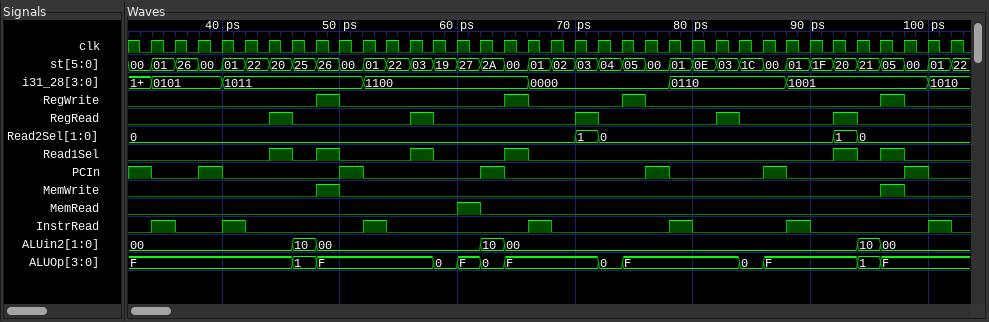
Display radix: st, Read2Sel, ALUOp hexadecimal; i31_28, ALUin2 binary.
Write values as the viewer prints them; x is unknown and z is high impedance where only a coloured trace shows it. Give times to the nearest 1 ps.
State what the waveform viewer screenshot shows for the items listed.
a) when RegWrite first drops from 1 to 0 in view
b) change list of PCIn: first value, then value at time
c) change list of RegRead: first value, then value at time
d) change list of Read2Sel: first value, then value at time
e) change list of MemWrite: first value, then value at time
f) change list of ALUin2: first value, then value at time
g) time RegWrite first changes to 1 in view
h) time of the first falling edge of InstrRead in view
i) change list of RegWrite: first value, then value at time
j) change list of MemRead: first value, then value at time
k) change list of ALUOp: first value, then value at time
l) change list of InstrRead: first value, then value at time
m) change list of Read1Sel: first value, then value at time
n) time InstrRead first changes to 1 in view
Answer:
50 ps
1, 0 at 34 ps, 1 at 38 ps, 0 at 40 ps, 1 at 50 ps, 0 at 52 ps, 1 at 62 ps, 0 at 64 ps, 1 at 76 ps, 0 at 78 ps, 1 at 86 ps, 0 at 88 ps, 1 at 98 ps, 0 at 100 ps
0, 1 at 44 ps, 0 at 46 ps, 1 at 56 ps, 0 at 58 ps, 1 at 70 ps, 0 at 72 ps, 1 at 82 ps, 0 at 84 ps, 1 at 92 ps, 0 at 94 ps
0, 1 at 70 ps, 0 at 72 ps, 1 at 92 ps, 0 at 94 ps
0, 1 at 48 ps, 0 at 50 ps, 1 at 96 ps, 0 at 98 ps
00, 10 at 46 ps, 00 at 48 ps, 10 at 62 ps, 00 at 64 ps, 10 at 94 ps, 00 at 96 ps
48 ps
36 ps
0, 1 at 48 ps, 0 at 50 ps, 1 at 64 ps, 0 at 66 ps, 1 at 74 ps, 0 at 76 ps, 1 at 96 ps, 0 at 98 ps
0, 1 at 60 ps, 0 at 62 ps
F, 1 at 46 ps, F at 48 ps, 0 at 58 ps, F at 60 ps, 0 at 62 ps, F at 64 ps, 0 at 72 ps, F at 74 ps, 0 at 84 ps, F at 86 ps, 1 at 94 ps, F at 96 ps
0, 1 at 34 ps, 0 at 36 ps, 1 at 40 ps, 0 at 42 ps, 1 at 52 ps, 0 at 54 ps, 1 at 66 ps, 0 at 68 ps, 1 at 78 ps, 0 at 80 ps, 1 at 88 ps, 0 at 90 ps, 1 at 100 ps, 0 at 102 ps
0, 1 at 44 ps, 0 at 46 ps, 1 at 48 ps, 0 at 50 ps, 1 at 56 ps, 0 at 58 ps, 1 at 64 ps, 0 at 66 ps, 1 at 92 ps, 0 at 94 ps, 1 at 96 ps, 0 at 98 ps
34 ps
